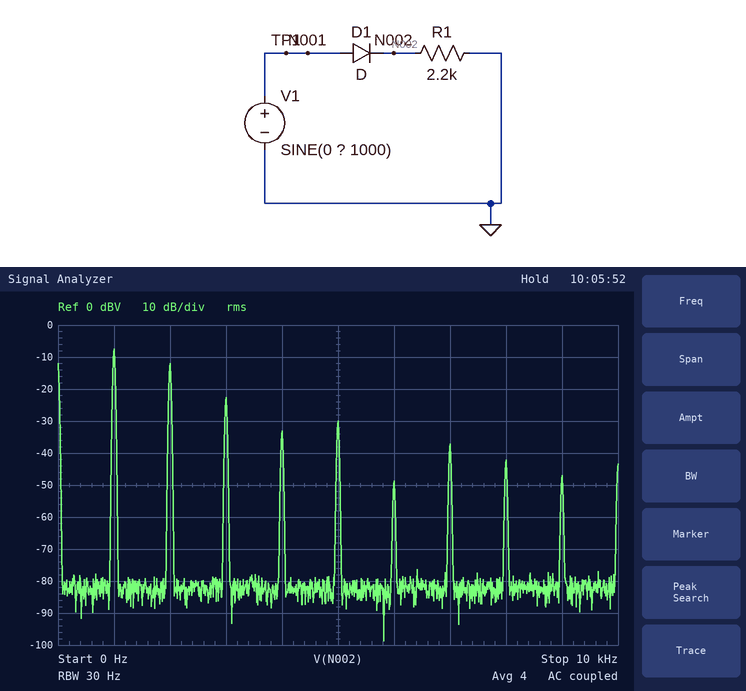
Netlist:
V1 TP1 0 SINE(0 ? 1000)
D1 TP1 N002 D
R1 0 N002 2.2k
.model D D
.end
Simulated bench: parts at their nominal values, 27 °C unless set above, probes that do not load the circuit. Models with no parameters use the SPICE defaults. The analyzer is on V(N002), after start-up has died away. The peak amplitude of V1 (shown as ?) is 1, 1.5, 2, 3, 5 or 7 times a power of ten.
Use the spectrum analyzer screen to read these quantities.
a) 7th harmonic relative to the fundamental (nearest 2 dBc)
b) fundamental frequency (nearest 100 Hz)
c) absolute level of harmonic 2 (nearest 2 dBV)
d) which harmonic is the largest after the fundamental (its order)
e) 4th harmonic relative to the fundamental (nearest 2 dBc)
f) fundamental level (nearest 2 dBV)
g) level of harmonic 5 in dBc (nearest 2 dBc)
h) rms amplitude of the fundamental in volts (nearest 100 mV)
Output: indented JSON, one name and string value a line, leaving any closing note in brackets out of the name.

{
  "7th harmonic relative to the fundamental": "-30 dBc",
  "fundamental frequency": "1.0 kHz",
  "absolute level of harmonic 2": "-12 dBV",
  "which harmonic is the largest after the fundamental": "2",
  "4th harmonic relative to the fundamental": "-26 dBc",
  "fundamental level": "-8 dBV",
  "level of harmonic 5 in dBc": "-22 dBc",
  "rms amplitude of the fundamental in volts": "400 mV"
}
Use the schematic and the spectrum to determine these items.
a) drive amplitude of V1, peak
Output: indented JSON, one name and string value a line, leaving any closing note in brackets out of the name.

{
  "drive amplitude of V1, peak": "2 V"
}
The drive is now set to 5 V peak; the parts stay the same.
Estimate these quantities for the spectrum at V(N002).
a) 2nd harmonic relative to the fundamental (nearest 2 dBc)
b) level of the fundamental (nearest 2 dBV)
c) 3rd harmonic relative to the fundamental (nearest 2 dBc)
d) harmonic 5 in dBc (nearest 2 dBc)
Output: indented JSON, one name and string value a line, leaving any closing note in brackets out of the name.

{
  "2nd harmonic relative to the fundamental": "-6 dBc",
  "level of the fundamental": "4 dBV",
  "3rd harmonic relative to the fundamental": "-24 dBc",
  "harmonic 5 in dBc": "-30 dBc"
}
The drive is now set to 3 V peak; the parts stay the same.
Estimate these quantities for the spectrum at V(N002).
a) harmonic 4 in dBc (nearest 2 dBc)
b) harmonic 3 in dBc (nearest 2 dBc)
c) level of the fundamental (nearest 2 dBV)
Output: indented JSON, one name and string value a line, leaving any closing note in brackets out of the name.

{
  "harmonic 4 in dBc": "-22 dBc",
  "harmonic 3 in dBc": "-20 dBc",
  "level of the fundamental": "-2 dBV"
}
